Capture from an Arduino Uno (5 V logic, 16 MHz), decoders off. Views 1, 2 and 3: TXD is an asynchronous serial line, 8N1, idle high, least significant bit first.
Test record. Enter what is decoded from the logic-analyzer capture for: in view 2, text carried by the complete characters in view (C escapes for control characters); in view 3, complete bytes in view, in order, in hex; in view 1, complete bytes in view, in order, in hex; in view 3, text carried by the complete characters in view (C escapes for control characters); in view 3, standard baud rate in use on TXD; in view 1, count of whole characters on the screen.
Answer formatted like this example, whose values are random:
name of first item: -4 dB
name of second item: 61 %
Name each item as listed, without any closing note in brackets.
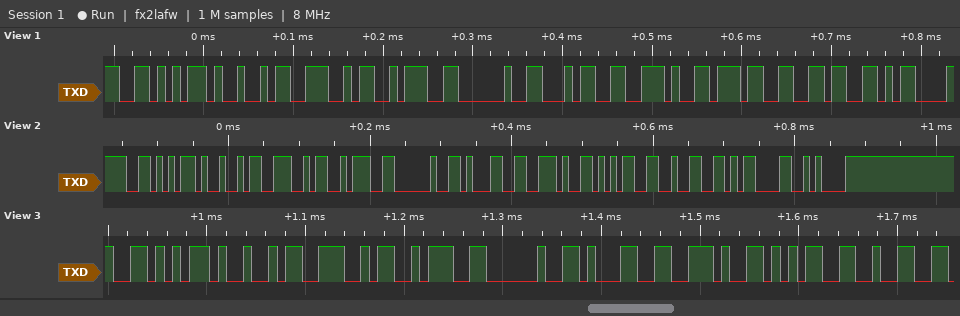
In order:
in view 2, text carried by the complete characters in view: "VIN: 1.52\r\n"
in view 3, complete bytes in view, in order, in hex: 56 49 4E 3A 20 31 2E 35 32
in view 1, complete bytes in view, in order, in hex: 0x56 0x49 0x4E 0x3A 0x20 0x34 0x2E 0x37 0x36 0x0D
in view 3, text carried by the complete characters in view: "VIN: 1.52"
in view 3, standard baud rate in use on TXD: 115200 baud
in view 1, count of whole characters on the screen: 10
